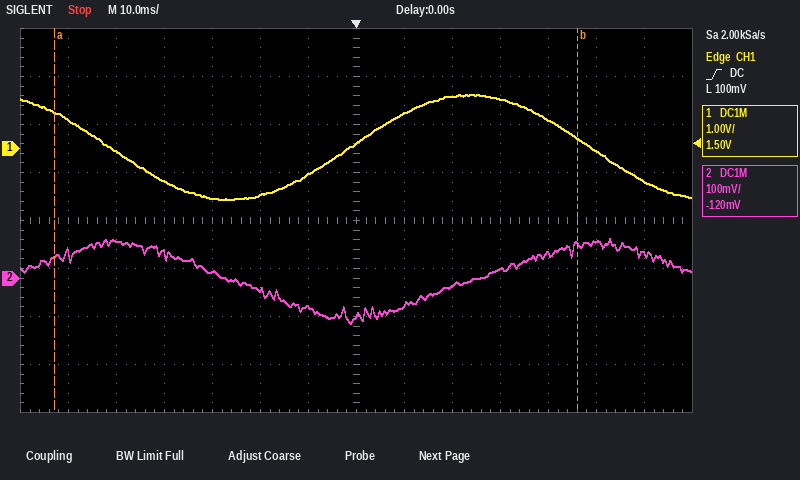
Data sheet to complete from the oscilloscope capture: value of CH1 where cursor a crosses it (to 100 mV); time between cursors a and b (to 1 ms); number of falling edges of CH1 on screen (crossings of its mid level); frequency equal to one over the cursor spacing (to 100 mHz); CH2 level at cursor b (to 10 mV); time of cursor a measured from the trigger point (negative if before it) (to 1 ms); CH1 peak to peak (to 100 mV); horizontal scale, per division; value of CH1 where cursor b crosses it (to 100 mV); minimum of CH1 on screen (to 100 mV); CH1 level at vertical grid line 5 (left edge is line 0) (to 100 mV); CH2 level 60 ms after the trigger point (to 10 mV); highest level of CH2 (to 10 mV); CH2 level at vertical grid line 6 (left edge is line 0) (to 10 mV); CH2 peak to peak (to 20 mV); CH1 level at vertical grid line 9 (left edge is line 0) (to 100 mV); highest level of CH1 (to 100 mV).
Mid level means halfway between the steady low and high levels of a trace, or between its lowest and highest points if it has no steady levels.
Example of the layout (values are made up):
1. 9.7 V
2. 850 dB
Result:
1. 800 mV
2. 109 ms
3. 2
4. 9.2 Hz
5. 70 mV
6. -63 ms
7. 2.2 V
8. 10 ms
9. 200 mV
10. -1.1 V
11. -1.0 V
12. 50 mV
13. 80 mV
14. -60 mV
15. 180 mV
16. 1.1 V
17. 1.1 V
